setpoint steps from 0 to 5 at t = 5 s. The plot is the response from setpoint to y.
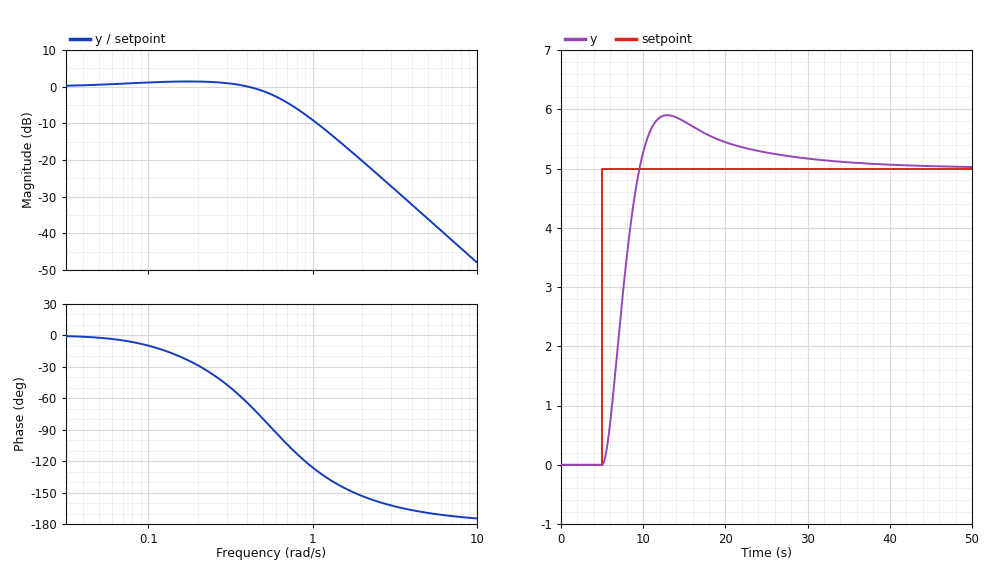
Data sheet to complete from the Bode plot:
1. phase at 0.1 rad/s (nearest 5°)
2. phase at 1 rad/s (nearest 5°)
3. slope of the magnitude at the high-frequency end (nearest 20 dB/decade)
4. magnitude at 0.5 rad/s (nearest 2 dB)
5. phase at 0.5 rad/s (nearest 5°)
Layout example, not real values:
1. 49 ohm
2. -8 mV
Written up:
1. -10°
2. -125°
3. -40 dB/decade
4. -2 dB
5. -80°
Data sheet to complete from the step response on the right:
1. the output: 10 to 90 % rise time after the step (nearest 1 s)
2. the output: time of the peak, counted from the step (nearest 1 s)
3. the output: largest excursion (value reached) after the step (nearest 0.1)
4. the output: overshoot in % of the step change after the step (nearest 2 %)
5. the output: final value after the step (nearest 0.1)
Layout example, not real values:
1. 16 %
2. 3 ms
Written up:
1. 3 s
2. 8 s
3. 5.9
4. 18 %
5. 5.0
